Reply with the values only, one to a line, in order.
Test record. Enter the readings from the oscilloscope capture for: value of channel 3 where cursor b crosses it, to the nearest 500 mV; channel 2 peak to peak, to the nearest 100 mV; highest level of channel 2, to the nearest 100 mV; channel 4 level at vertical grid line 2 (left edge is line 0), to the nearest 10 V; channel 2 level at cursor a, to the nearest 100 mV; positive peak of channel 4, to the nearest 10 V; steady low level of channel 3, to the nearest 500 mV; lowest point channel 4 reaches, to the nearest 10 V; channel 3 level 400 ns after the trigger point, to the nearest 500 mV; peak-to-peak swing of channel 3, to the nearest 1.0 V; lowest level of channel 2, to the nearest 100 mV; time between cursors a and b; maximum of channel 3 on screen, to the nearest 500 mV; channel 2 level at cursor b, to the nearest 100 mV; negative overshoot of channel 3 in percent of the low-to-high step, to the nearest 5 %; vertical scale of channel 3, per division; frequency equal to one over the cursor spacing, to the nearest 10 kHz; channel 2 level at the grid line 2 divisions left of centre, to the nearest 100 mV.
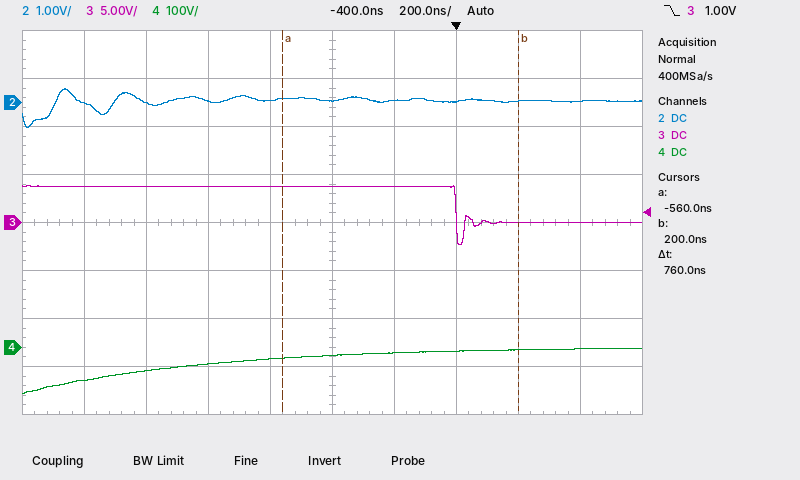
0.0 V
800 mV
300 mV
-50 V
100 mV
0 V
0.0 V
-100 V
0.0 V
6.0 V
-500 mV
760 ns
4.0 V
0.0 V
60 %
5 V
1.32 MHz
0.0 V
